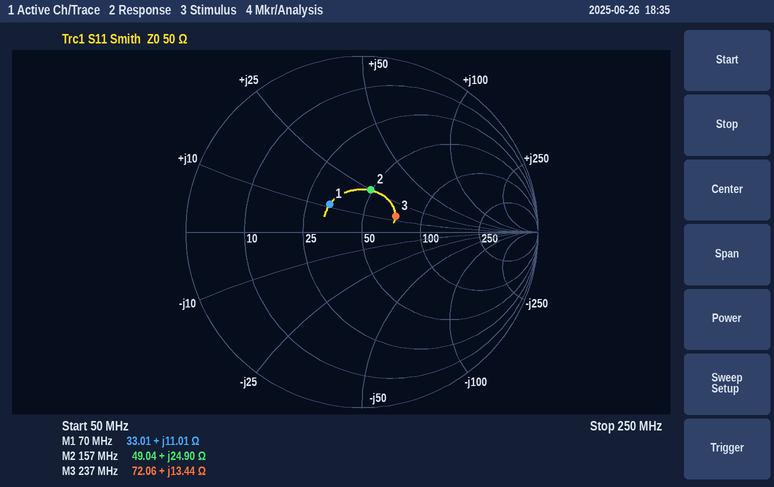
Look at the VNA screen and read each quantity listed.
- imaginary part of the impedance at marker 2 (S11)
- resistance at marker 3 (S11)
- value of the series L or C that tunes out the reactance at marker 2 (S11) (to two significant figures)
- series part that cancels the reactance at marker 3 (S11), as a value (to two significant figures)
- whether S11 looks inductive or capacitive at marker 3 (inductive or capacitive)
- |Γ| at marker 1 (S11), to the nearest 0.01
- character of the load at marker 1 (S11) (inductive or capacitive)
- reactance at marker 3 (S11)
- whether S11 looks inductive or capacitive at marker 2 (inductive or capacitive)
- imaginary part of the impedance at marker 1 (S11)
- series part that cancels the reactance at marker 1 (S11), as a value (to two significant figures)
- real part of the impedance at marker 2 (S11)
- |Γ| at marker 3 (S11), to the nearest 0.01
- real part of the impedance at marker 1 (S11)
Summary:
+24.90 Ω
72.06 Ω
41 pF
50 pF
inductive
0.24
inductive
+13.44 Ω
inductive
+11.01 Ω
210 pF
49.04 Ω
0.21
33.01 Ω
